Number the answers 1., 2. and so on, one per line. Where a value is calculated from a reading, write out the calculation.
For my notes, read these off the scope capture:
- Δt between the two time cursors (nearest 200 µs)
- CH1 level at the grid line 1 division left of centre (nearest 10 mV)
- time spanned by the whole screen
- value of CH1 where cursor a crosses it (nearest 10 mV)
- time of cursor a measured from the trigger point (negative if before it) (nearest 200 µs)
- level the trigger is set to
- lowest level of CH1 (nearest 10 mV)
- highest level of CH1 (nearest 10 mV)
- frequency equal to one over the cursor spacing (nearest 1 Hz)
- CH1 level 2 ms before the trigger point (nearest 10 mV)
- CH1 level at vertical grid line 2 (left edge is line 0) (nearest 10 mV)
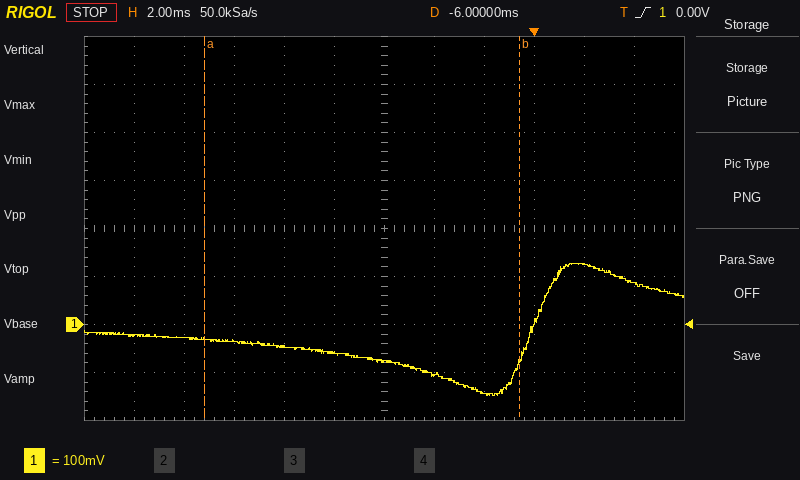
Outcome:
1. 12.6 ms
2. -60 mV
3. 24 ms
4. -30 mV
5. -13.2 ms
6. 0.00 V
7. -150 mV
8. 130 mV
9. 1 / 12.6 ms ≈ 79 Hz
10. -140 mV
11. -30 mV
